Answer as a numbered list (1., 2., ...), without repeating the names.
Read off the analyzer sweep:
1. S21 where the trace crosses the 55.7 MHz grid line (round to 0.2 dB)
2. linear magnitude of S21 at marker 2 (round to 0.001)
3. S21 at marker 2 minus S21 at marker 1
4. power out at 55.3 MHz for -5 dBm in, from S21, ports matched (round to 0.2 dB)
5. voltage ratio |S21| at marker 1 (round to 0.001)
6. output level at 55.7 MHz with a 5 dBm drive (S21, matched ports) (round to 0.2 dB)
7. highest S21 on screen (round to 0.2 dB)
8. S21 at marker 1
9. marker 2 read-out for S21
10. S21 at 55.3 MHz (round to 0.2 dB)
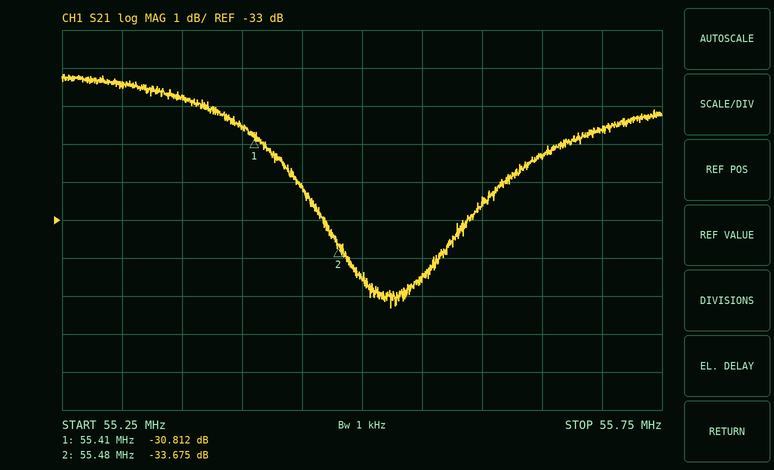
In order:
1. -30.6 dB
2. 0.021
3. -2.863 dB
4. -34.4 dBm
5. 0.029
6. -25.6 dBm
7. -29.2 dB
8. -30.812 dB
9. -33.675 dB
10. -29.4 dB
